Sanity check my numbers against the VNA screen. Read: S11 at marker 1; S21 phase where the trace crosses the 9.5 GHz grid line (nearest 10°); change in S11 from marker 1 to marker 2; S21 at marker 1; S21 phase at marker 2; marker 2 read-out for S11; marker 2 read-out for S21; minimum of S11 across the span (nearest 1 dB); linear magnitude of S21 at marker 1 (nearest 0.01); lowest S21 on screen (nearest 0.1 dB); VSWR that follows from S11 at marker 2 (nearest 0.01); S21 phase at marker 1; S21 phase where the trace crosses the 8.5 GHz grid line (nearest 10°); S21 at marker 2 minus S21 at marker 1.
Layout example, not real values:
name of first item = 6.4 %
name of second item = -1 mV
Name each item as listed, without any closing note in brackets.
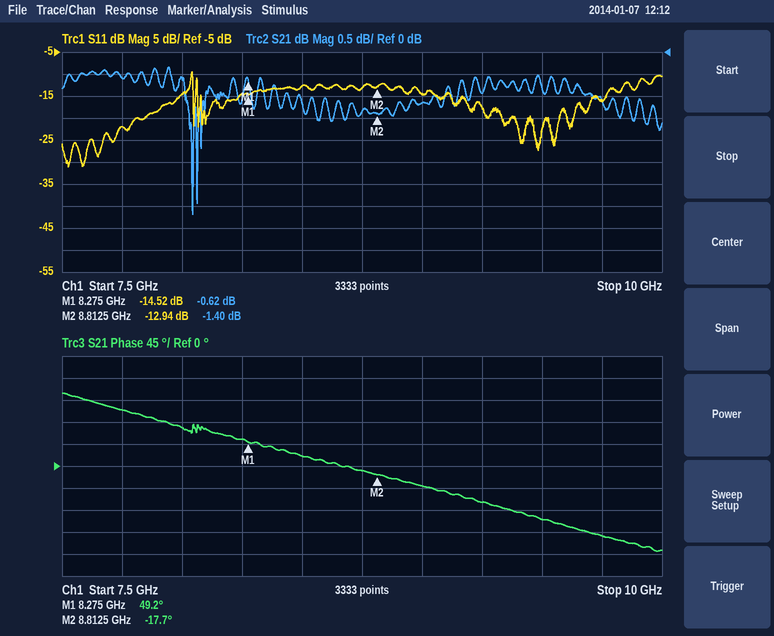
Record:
S11 at marker 1 = -14.52 dB
S21 phase where the trace crosses the 9.5 GHz grid line = -110°
change in S11 from marker 1 to marker 2 = 1.58 dB
S21 at marker 1 = -0.62 dB
S21 phase at marker 2 = -17.7°
marker 2 read-out for S11 = -12.94 dB
marker 2 read-out for S21 = -1.40 dB
minimum of S11 across the span = -31 dB
linear magnitude of S21 at marker 1 = 0.93
lowest S21 on screen = -3.7 dB
VSWR that follows from S11 at marker 2 = 1.58
S21 phase at marker 1 = 49.2°
S21 phase where the trace crosses the 8.5 GHz grid line = 20°
S21 at marker 2 minus S21 at marker 1 = -0.78 dB
